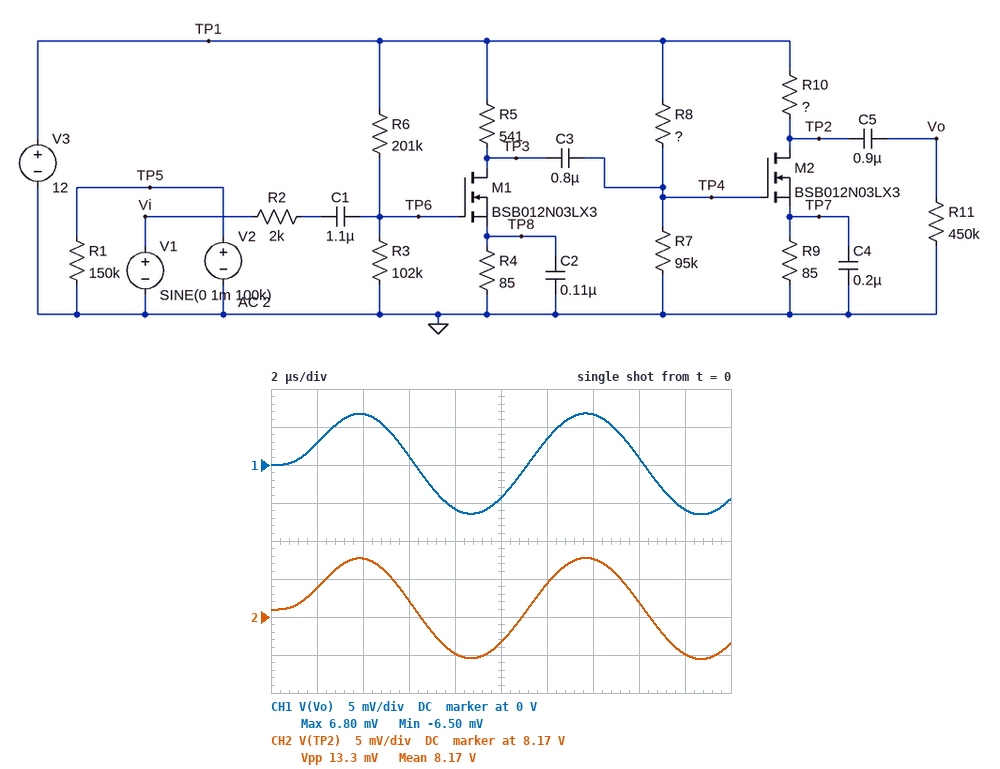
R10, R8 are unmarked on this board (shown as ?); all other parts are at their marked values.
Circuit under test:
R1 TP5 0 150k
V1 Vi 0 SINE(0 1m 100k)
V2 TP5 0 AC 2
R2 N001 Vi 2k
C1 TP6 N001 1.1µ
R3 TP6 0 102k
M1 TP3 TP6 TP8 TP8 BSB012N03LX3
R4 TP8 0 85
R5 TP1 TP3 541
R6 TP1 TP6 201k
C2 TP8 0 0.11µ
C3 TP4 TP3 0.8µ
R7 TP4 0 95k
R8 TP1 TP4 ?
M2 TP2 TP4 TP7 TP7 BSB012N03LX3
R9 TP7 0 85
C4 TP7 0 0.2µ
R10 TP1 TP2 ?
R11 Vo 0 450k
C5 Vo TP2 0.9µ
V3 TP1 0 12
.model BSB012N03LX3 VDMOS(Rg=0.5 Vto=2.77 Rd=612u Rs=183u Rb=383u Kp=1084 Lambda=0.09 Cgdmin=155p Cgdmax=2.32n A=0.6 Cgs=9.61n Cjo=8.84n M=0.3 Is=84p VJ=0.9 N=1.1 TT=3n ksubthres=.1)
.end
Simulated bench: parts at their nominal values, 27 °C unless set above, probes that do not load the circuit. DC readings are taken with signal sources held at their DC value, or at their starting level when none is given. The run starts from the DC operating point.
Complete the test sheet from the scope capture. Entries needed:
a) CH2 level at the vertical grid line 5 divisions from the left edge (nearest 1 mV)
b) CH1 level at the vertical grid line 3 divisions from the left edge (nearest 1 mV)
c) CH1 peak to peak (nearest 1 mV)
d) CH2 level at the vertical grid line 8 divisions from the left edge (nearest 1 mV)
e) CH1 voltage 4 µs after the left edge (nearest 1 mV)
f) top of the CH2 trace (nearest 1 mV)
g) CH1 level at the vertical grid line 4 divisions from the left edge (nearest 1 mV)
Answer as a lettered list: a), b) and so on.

a) 8.167 V
b) 1 mV
c) 13 mV
d) 8.172 V
e) 7 mV
f) 8.178 V
g) -6 mV
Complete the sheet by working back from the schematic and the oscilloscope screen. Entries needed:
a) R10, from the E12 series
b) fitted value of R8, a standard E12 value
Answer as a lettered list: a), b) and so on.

a) 150 Ω
b) 150 kΩ
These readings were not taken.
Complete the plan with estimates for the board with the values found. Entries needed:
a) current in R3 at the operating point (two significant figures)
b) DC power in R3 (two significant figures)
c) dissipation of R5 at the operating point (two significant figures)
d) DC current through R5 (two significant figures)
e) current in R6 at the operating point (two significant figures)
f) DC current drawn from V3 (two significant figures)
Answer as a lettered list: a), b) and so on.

a) 40 µA
b) 160 µW
c) 180 mW
d) 18 mA
e) 40 µA
f) 44 mA
